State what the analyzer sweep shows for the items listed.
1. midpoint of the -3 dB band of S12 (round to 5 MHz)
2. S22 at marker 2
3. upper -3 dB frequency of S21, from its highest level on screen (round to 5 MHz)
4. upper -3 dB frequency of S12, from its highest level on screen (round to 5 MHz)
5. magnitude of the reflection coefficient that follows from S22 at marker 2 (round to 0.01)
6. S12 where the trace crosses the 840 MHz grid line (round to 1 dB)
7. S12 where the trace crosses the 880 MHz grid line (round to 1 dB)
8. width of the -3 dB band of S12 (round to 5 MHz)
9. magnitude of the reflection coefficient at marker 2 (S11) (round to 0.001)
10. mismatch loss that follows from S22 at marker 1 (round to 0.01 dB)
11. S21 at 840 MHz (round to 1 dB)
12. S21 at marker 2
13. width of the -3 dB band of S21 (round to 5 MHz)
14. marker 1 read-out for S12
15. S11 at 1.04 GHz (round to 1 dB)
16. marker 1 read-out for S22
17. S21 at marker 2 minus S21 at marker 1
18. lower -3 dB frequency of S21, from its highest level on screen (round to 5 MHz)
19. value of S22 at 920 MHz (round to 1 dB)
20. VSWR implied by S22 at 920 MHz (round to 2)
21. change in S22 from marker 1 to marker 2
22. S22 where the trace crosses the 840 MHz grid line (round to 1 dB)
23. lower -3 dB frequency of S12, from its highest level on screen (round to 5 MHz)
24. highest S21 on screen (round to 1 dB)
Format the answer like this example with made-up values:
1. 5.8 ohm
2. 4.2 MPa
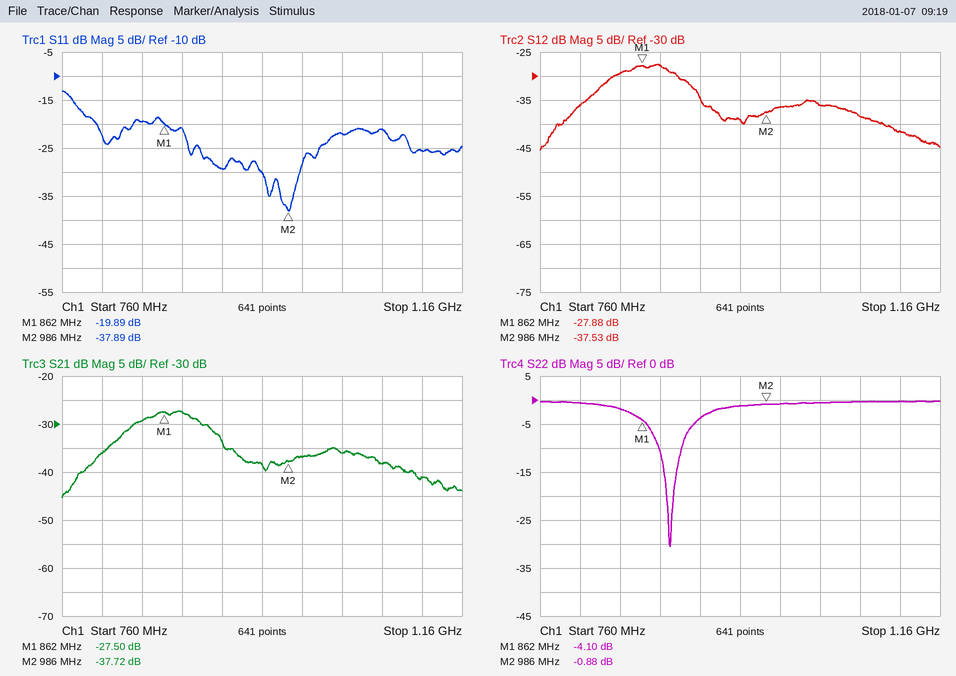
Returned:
1. 865 MHz
2. -0.88 dB
3. 905 MHz
4. 900 MHz
5. 0.90
6. -29 dB
7. -28 dB
8. 70 MHz
9. 0.013
10. 2.14 dB
11. -29 dB
12. -37.72 dB
13. 75 MHz
14. -27.88 dB
15. -22 dB
16. -4.10 dB
17. -10.22 dB
18. 830 MHz
19. -4 dB
20. 4
21. 3.22 dB
22. -2 dB
23. 830 MHz
24. -27 dB
